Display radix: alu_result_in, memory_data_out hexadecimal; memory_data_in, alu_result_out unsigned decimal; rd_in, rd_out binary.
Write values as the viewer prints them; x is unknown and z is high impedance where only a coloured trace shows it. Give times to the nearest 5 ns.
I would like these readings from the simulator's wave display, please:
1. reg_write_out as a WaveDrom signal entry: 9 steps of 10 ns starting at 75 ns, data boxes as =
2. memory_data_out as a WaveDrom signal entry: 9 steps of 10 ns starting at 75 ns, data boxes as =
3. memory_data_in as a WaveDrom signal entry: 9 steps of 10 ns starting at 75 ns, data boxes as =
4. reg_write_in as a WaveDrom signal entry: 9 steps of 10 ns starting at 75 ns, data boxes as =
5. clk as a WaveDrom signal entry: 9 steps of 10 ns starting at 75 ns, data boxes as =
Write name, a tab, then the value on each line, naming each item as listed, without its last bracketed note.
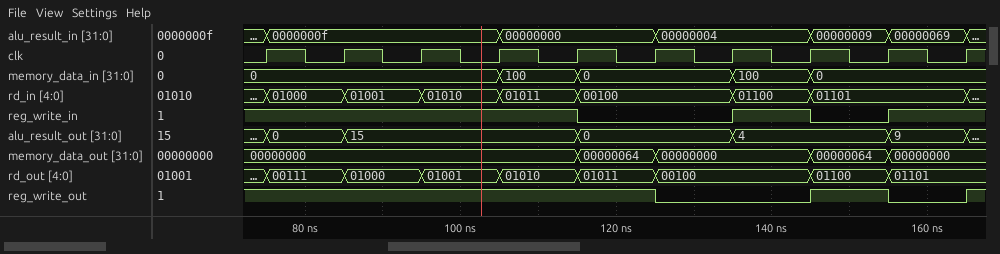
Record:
reg_write_out as a WaveDrom signal entry: 9 steps of 10 ns starting at 75 ns, data boxes as =	{name: 'reg_write_out', wave: '1....0.10'}
memory_data_out as a WaveDrom signal entry: 9 steps of 10 ns starting at 75 ns, data boxes as =	{name: 'memory_data_out', wave: '=...==.==', data: '00000000 00000064 00000000 00000064 00000000'}
memory_data_in as a WaveDrom signal entry: 9 steps of 10 ns starting at 75 ns, data boxes as =	{name: 'memory_data_in', wave: '=..==.==.', data: '0 100 0 100 0'}
reg_write_in as a WaveDrom signal entry: 9 steps of 10 ns starting at 75 ns, data boxes as =	{name: 'reg_write_in', wave: '1...0.101'}
clk as a WaveDrom signal entry: 9 steps of 10 ns starting at 75 ns, data boxes as =	{name: 'clk', wave: 'p........'}
